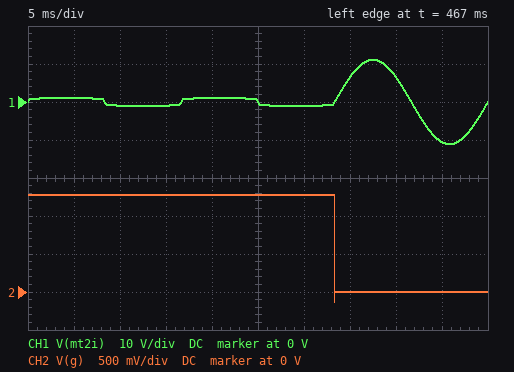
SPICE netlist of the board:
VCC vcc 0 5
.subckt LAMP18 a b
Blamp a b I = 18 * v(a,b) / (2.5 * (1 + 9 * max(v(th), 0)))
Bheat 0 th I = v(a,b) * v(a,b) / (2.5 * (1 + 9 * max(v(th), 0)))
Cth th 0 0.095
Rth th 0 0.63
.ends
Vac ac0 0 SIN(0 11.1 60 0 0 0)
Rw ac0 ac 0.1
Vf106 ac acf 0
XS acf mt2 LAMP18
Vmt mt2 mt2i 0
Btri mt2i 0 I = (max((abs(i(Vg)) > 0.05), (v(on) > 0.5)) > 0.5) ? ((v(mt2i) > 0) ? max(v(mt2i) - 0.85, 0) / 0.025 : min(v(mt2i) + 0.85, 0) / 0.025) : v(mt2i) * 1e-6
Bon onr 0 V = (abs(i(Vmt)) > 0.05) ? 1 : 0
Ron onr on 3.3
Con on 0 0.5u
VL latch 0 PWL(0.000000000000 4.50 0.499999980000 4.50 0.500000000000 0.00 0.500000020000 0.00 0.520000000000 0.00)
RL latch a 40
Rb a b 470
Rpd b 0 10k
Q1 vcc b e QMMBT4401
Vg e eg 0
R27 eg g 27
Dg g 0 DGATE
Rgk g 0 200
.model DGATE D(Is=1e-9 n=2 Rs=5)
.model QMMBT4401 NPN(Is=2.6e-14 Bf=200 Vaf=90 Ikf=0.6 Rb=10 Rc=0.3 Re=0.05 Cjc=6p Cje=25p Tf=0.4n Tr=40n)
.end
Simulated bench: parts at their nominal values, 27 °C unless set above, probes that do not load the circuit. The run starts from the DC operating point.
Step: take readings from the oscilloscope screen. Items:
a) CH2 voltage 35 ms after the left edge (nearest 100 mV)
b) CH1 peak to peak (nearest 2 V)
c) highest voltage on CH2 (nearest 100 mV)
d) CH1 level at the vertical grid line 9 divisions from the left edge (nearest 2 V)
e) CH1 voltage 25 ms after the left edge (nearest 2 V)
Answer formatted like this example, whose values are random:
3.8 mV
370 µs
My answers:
0 V
22 V
1.3 V
-10 V
0 V
